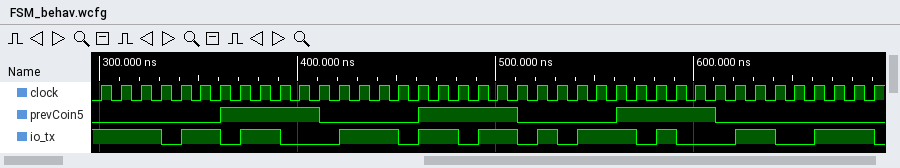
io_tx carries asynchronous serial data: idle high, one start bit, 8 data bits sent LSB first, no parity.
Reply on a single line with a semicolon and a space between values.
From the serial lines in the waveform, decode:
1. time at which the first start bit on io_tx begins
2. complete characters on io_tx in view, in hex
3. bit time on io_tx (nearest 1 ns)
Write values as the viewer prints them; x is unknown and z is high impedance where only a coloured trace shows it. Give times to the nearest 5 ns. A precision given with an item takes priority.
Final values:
330 ns; 1B, 5B, 31; 10 ns
